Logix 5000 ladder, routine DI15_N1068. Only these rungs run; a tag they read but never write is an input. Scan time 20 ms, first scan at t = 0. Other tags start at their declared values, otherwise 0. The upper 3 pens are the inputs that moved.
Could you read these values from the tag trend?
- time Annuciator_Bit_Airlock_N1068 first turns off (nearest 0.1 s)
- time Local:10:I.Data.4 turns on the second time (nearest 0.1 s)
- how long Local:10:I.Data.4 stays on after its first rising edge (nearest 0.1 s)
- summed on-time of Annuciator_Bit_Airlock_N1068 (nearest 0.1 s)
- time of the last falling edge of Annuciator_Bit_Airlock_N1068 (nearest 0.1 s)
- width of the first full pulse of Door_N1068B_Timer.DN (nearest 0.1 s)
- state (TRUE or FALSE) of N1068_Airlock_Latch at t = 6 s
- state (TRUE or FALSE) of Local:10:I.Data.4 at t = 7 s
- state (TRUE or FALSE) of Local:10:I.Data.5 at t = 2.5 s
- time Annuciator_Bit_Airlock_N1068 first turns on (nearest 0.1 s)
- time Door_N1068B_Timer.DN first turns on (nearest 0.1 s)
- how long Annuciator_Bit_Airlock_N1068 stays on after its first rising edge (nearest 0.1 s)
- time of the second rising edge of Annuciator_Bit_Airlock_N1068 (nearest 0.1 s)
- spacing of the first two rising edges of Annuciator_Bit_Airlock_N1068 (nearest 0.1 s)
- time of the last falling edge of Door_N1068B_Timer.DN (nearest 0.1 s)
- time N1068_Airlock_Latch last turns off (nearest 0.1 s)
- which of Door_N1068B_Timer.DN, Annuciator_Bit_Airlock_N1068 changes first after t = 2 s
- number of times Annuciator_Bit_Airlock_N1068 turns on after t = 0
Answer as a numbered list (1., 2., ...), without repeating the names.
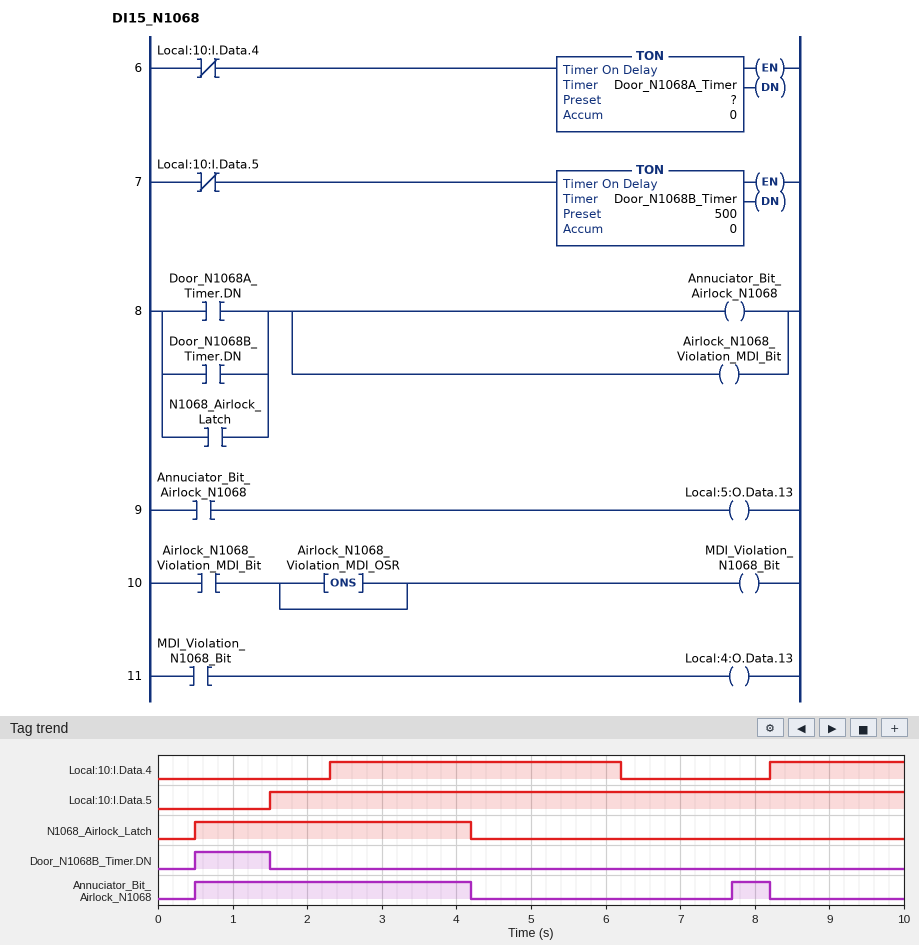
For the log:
1. 4.2 s
2. 8.2 s
3. 3.9 s
4. 4.2 s
5. 8.2 s
6. 1.0 s
7. FALSE
8. FALSE
9. TRUE
10. 0.5 s
11. 0.5 s
12. 3.7 s
13. 7.7 s
14. 7.2 s
15. 1.5 s
16. 4.2 s
17. Annuciator_Bit_Airlock_N1068
18. 2
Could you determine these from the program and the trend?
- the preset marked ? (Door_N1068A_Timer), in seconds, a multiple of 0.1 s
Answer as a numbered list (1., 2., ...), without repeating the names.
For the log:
1. 1.5 s
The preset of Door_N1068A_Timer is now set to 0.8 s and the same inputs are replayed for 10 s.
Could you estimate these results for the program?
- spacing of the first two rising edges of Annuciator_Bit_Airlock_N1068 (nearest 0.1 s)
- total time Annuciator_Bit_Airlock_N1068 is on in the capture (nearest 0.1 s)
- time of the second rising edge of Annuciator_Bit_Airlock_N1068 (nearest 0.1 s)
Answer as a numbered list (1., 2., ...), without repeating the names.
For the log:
1. 6.5 s
2. 4.9 s
3. 7.0 s
